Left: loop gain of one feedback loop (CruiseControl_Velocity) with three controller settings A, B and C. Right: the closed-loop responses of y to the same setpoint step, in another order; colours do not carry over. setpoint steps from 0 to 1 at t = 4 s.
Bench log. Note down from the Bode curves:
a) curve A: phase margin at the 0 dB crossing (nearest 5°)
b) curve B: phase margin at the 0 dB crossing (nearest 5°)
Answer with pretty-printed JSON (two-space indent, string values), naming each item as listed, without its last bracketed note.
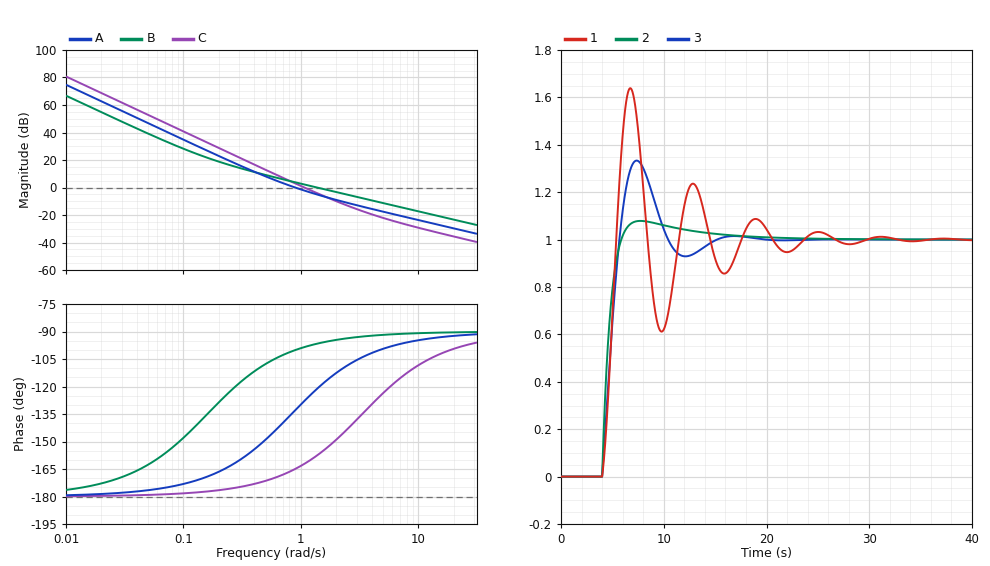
{
  "curve A: phase margin at the 0 dB crossing": "45°",
  "curve B: phase margin at the 0 dB crossing": "85°"
}
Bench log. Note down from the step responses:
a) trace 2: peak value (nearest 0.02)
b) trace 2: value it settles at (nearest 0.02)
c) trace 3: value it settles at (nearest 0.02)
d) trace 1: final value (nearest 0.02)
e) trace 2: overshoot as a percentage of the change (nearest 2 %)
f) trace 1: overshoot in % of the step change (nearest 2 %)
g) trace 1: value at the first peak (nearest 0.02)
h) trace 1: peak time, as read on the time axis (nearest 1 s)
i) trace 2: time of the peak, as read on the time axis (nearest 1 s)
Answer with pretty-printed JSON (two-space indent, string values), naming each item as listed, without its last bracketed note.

{
  "trace 2: peak value": "1.08",
  "trace 2: value it settles at": "1.00",
  "trace 3: value it settles at": "1.00",
  "trace 1: final value": "1.00",
  "trace 2: overshoot as a percentage of the change": "8 %",
  "trace 1: overshoot in % of the step change": "64 %",
  "trace 1: value at the first peak": "1.64",
  "trace 1: peak time, as read on the time axis": "7 s",
  "trace 2: time of the peak, as read on the time axis": "8 s"
}
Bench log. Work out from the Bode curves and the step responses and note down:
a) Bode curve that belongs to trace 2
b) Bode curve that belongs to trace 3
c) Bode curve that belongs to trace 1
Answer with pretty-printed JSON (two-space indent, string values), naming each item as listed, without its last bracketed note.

{
  "Bode curve that belongs to trace 2": "B",
  "Bode curve that belongs to trace 3": "A",
  "Bode curve that belongs to trace 1": "C"
}
